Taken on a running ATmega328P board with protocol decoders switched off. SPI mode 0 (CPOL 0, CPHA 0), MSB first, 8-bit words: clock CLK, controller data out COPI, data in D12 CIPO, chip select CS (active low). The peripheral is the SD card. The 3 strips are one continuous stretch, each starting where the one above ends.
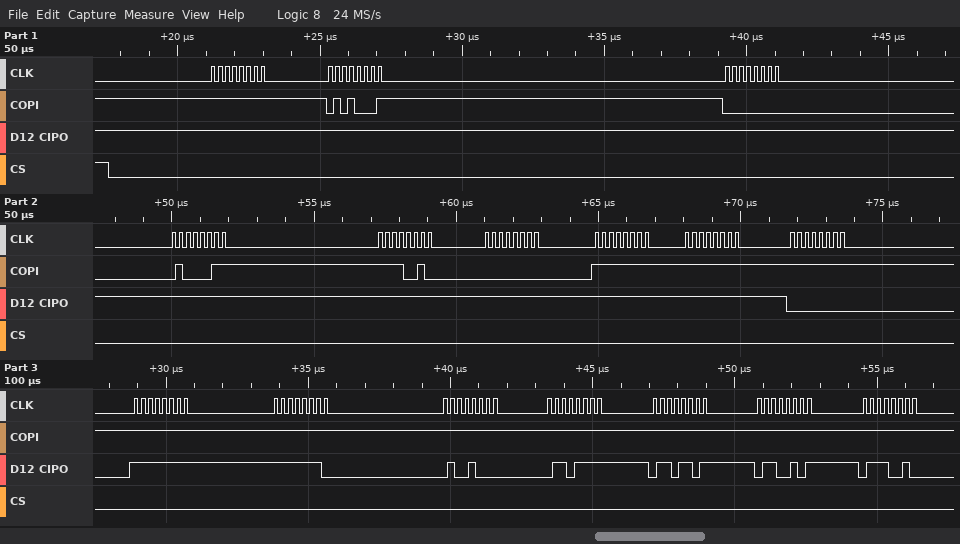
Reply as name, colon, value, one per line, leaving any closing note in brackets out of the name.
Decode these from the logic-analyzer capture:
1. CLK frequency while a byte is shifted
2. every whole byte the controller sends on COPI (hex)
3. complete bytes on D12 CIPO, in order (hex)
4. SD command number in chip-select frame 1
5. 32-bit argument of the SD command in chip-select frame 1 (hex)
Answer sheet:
CLK frequency while a byte is shifted: 4 MHz
every whole byte the controller sends on COPI: FF 51 00 43 F2 00 FF FF FF FF FF FF FF FF FF FF
complete bytes on D12 CIPO, in order: FF FF FF FF FF FF FF FF 00 FF FE 48 6F 6D 65 72
SD command number in chip-select frame 1: CMD17
32-bit argument of the SD command in chip-select frame 1: 0x0043F200
